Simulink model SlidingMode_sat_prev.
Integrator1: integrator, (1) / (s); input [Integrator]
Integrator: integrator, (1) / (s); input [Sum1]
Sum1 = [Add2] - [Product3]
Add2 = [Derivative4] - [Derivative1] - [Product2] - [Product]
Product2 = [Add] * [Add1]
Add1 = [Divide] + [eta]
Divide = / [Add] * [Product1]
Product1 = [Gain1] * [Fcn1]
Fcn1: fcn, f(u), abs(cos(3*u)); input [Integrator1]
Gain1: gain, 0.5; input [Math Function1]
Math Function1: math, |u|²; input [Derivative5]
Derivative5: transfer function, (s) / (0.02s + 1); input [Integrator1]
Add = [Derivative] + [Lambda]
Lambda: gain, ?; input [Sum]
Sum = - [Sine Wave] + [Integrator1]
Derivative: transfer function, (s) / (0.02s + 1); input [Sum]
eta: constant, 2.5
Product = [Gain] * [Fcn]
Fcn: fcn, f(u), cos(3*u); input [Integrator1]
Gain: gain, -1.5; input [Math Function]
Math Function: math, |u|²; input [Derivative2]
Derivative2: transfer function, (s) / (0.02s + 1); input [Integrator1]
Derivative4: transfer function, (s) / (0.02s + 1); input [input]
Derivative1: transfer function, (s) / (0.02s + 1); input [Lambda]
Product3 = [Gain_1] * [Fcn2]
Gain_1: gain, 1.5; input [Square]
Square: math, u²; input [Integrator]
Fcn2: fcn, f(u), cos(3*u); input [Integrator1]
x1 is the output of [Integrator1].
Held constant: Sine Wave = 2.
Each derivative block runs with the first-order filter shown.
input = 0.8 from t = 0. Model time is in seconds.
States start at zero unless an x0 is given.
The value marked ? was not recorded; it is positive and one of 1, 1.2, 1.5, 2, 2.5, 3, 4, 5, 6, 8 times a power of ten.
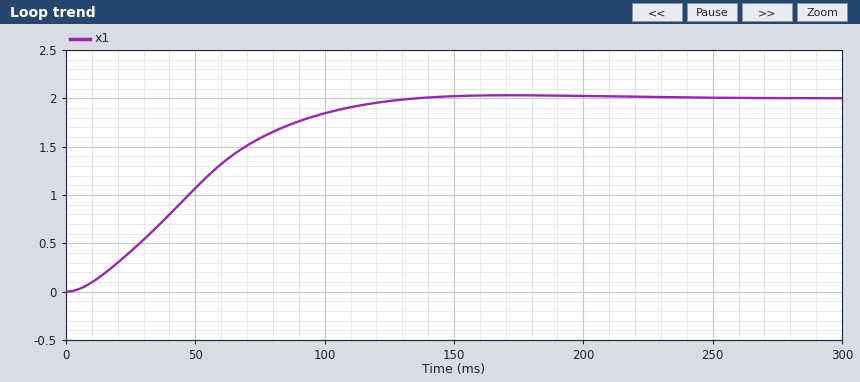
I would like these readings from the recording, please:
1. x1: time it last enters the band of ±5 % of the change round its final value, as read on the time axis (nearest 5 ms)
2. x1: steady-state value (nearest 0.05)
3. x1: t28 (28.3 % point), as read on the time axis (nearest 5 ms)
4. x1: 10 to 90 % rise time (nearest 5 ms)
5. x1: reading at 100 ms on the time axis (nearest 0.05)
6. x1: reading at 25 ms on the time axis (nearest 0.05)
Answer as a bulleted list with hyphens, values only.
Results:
- 110 ms
- 2.00
- 30 ms
- 80 ms
- 1.85
- 0.40
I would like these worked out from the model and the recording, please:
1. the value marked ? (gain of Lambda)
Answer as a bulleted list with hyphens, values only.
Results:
- 20
